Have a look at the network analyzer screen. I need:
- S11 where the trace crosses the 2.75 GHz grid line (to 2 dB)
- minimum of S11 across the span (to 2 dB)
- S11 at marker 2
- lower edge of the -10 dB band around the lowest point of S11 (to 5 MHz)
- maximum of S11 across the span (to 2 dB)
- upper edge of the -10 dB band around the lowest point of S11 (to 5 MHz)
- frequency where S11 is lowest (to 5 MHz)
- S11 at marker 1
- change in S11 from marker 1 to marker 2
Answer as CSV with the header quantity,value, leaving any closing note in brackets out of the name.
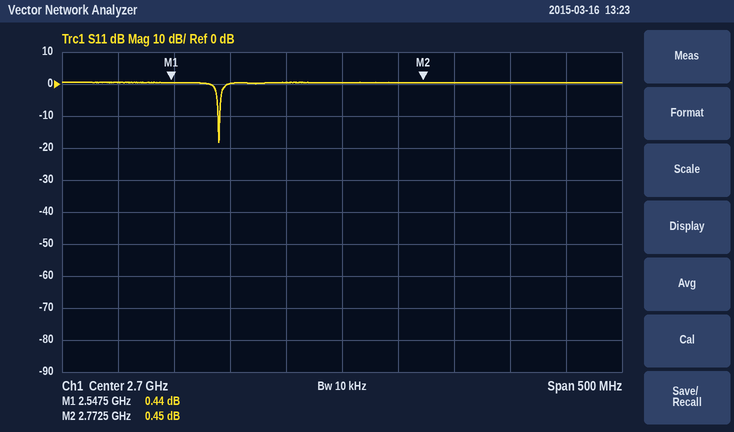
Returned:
quantity,value
S11 where the trace crosses the 2.75 GHz grid line,0 dB
minimum of S11 across the span,-18 dB
S11 at marker 2,0.45 dB
lower edge of the -10 dB band around the lowest point of S11,2.590 GHz
maximum of S11 across the span,0 dB
upper edge of the -10 dB band around the lowest point of S11,2.590 GHz
frequency where S11 is lowest,2.590 GHz
S11 at marker 1,0.44 dB
change in S11 from marker 1 to marker 2,0.01 dB
